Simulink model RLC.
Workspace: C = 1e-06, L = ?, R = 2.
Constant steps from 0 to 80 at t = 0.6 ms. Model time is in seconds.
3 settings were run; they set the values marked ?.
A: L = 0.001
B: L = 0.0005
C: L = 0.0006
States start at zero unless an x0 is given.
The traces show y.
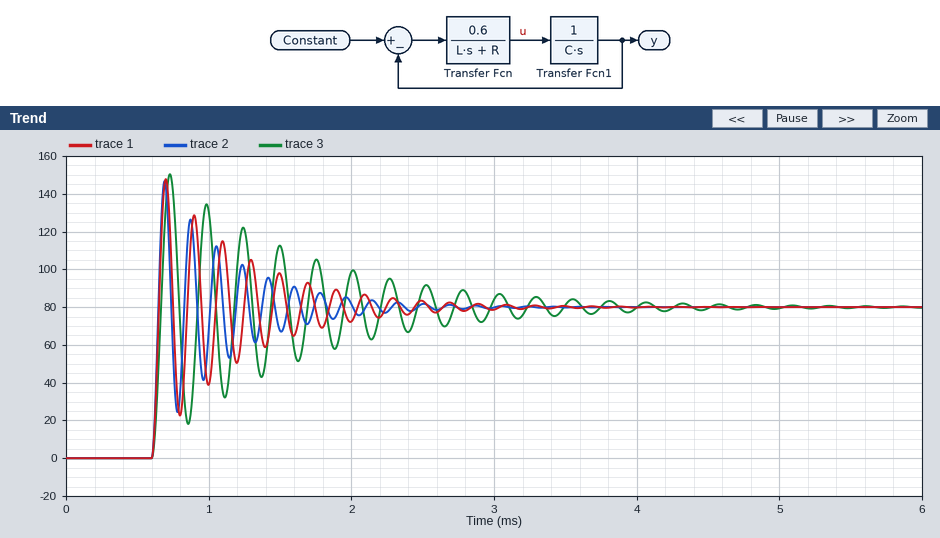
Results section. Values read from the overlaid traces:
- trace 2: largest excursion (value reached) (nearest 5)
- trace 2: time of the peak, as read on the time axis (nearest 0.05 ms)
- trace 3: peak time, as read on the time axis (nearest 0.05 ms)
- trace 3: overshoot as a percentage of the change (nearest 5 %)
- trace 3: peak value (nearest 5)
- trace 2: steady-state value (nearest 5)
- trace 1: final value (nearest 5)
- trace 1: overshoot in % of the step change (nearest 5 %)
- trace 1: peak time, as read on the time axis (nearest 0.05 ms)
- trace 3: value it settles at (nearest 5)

145
0.70 ms
0.75 ms
90 %
150
80
80
85 %
0.70 ms
80
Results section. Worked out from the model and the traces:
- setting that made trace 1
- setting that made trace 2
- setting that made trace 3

C
B
A
